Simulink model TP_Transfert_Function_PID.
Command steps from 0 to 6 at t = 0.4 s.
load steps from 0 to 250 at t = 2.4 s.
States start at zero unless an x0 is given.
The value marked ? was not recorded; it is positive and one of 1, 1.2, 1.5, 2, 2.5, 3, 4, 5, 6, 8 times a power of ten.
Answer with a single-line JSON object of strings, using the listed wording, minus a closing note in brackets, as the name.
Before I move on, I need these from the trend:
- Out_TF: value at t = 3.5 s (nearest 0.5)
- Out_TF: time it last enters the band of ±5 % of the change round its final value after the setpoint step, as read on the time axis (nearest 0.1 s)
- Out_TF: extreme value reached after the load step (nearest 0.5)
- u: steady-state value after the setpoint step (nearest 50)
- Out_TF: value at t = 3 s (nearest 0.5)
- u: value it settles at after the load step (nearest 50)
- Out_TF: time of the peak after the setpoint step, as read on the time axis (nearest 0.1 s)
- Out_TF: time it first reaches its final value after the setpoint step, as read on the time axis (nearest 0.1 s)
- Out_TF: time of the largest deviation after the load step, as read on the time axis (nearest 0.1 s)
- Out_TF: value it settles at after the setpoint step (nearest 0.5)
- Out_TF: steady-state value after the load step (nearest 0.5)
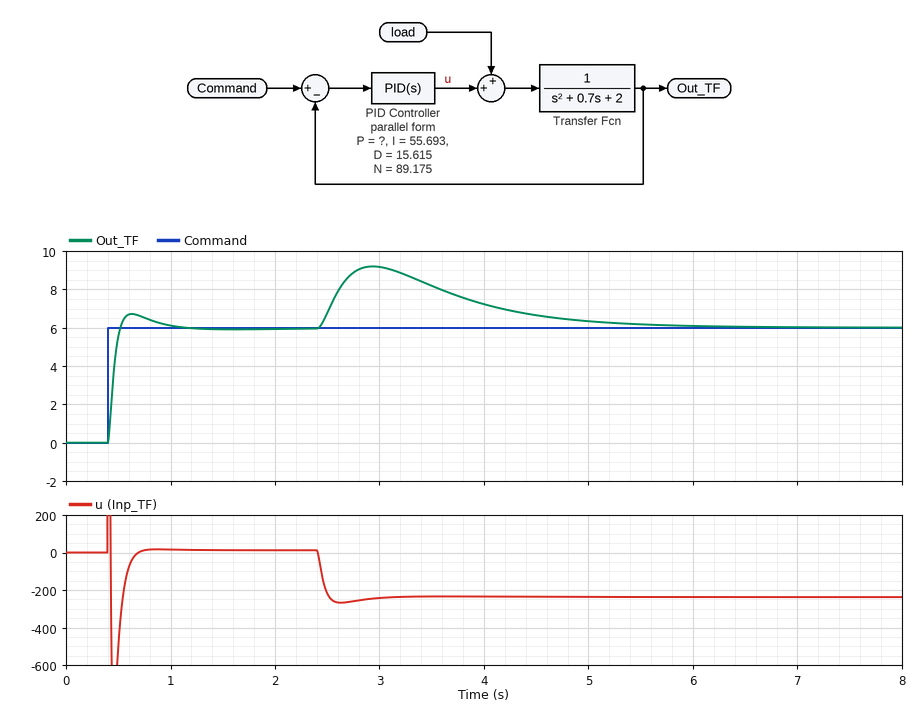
{"Out_TF: value at t = 3.5 s": "8.0", "Out_TF: time it last enters the band of ±5 % of the change round its final value after the setpoint step, as read on the time axis": "0.9 s", "Out_TF: extreme value reached after the load step": "9.0", "u: steady-state value after the setpoint step": "0", "Out_TF: value at t = 3 s": "9.0", "u: value it settles at after the load step": "-250", "Out_TF: time of the peak after the setpoint step, as read on the time axis": "0.6 s", "Out_TF: time it first reaches its final value after the setpoint step, as read on the time axis": "0.5 s", "Out_TF: time of the largest deviation after the load step, as read on the time axis": "2.9 s", "Out_TF: value it settles at after the setpoint step": "6.0", "Out_TF: steady-state value after the load step": "6.0"}
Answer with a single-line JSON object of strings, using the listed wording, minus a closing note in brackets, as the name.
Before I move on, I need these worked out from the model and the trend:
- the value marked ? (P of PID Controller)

{"the value marked ?": "60"}
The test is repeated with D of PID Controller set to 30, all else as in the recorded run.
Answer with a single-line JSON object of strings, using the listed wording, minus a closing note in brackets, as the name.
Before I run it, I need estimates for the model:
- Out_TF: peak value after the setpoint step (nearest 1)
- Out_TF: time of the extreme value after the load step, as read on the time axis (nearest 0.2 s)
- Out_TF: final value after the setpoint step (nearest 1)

{"Out_TF: peak value after the setpoint step": "6", "Out_TF: time of the extreme value after the load step, as read on the time axis": "3.2 s", "Out_TF: final value after the setpoint step": "6"}
